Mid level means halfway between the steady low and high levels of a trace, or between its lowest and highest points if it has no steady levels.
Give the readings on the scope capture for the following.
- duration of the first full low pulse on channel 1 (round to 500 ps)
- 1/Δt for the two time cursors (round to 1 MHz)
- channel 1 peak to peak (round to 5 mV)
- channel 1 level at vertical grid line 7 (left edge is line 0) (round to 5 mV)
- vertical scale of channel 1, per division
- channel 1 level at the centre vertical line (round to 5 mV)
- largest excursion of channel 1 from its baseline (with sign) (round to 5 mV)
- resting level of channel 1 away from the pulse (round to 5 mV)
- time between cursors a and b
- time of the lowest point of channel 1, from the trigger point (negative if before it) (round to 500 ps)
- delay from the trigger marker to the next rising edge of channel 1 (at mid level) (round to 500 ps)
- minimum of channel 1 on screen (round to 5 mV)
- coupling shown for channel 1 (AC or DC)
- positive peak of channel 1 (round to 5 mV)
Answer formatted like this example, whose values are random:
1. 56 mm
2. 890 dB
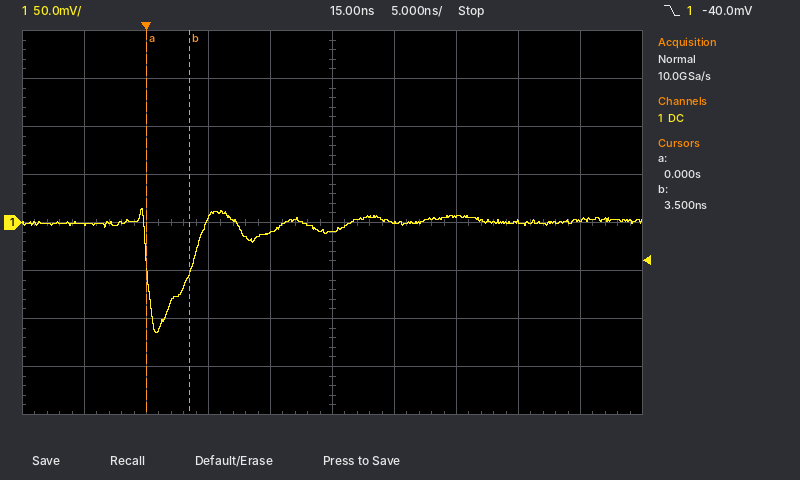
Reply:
1. 3.5 ns
2. 286 MHz
3. 130 mV
4. 5 mV
5. 50 mV
6. -10 mV
7. -115 mV
8. 0 mV
9. 3.5 ns
10. +1.0 ns
11. 3.5 ns
12. -115 mV
13. DC
14. 15 mV
